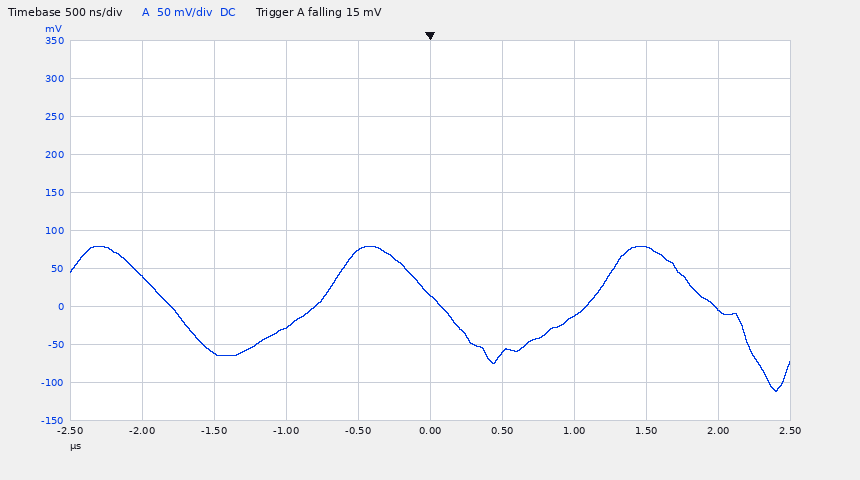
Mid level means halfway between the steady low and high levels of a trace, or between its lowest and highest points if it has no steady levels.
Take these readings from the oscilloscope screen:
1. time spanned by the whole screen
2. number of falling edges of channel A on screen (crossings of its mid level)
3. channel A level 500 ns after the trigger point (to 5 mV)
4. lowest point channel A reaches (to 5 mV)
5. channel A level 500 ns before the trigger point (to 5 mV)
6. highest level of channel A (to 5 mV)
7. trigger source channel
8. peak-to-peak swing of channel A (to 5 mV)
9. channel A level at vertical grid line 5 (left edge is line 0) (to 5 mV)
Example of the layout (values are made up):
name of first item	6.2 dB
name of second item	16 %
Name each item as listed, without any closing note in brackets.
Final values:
time spanned by the whole screen	5 µs
number of falling edges of channel A on screen	3
channel A level 500 ns after the trigger point	-60 mV
lowest point channel A reaches	-110 mV
channel A level 500 ns before the trigger point	75 mV
highest level of channel A	80 mV
trigger source channel	channel A
peak-to-peak swing of channel A	190 mV
channel A level at vertical grid line 5 (left edge is line 0)	15 mV
